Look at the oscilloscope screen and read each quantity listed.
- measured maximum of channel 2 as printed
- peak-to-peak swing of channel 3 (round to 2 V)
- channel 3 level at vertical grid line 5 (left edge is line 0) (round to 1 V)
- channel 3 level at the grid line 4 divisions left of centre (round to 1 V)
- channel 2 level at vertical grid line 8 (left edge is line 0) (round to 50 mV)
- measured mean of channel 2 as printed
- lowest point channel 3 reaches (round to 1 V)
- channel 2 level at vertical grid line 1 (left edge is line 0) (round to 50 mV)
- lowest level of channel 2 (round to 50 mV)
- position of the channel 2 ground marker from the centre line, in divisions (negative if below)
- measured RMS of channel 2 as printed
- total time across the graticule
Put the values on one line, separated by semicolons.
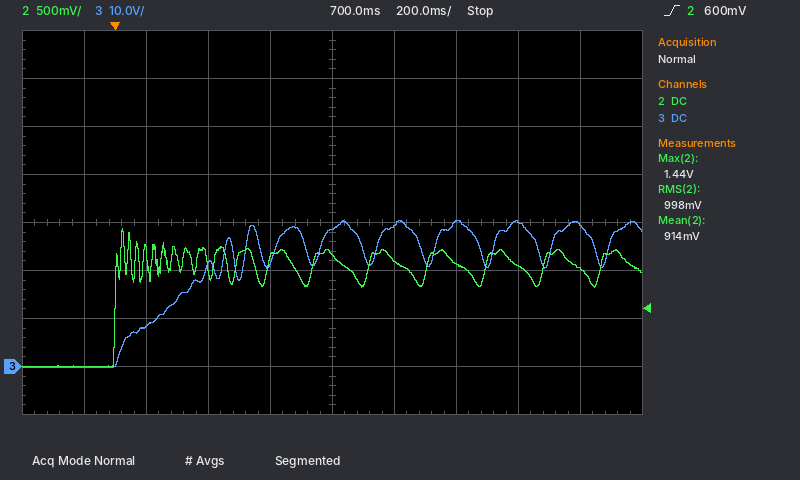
1.44 V; 30 V; 29 V; 0 V; 1.05 V; 914 mV; 0 V; 0 mV; 0 mV; -3.0 div; 998 mV; 2 s
